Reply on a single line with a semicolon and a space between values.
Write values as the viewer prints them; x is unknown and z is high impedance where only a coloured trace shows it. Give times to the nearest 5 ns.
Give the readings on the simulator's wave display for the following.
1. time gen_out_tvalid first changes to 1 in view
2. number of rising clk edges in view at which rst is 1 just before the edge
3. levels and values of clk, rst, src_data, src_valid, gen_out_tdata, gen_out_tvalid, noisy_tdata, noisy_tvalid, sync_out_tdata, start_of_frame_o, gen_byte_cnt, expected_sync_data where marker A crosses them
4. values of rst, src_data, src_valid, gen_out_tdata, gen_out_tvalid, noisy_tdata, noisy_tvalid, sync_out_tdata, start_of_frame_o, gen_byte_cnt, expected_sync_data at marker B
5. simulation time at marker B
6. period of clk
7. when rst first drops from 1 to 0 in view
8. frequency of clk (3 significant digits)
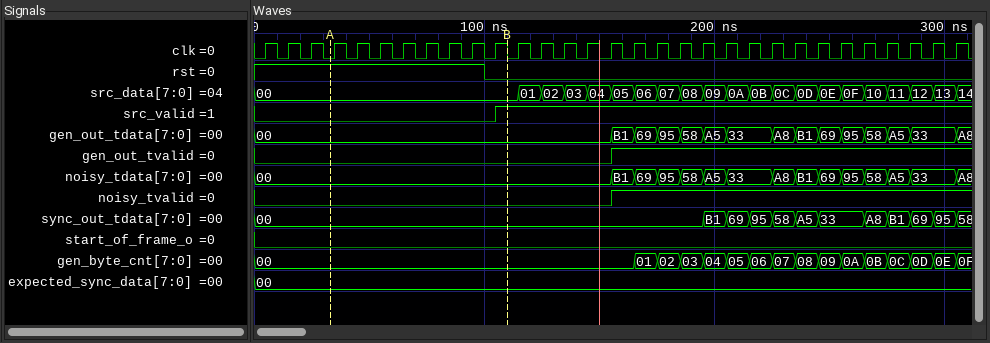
155 ns; 10; clk=0, rst=1, src_data=00, src_valid=0, gen_out_tdata=00, gen_out_tvalid=0, noisy_tdata=00, noisy_tvalid=0, sync_out_tdata=00, start_of_frame_o=0, gen_byte_cnt=00, expected_sync_data=00; rst=0, src_data=00, src_valid=1, gen_out_tdata=00, gen_out_tvalid=0, noisy_tdata=00, noisy_tvalid=0, sync_out_tdata=00, start_of_frame_o=0, gen_byte_cnt=00, expected_sync_data=00; 110 ns; 10 ns; 100 ns; 100 MHz
